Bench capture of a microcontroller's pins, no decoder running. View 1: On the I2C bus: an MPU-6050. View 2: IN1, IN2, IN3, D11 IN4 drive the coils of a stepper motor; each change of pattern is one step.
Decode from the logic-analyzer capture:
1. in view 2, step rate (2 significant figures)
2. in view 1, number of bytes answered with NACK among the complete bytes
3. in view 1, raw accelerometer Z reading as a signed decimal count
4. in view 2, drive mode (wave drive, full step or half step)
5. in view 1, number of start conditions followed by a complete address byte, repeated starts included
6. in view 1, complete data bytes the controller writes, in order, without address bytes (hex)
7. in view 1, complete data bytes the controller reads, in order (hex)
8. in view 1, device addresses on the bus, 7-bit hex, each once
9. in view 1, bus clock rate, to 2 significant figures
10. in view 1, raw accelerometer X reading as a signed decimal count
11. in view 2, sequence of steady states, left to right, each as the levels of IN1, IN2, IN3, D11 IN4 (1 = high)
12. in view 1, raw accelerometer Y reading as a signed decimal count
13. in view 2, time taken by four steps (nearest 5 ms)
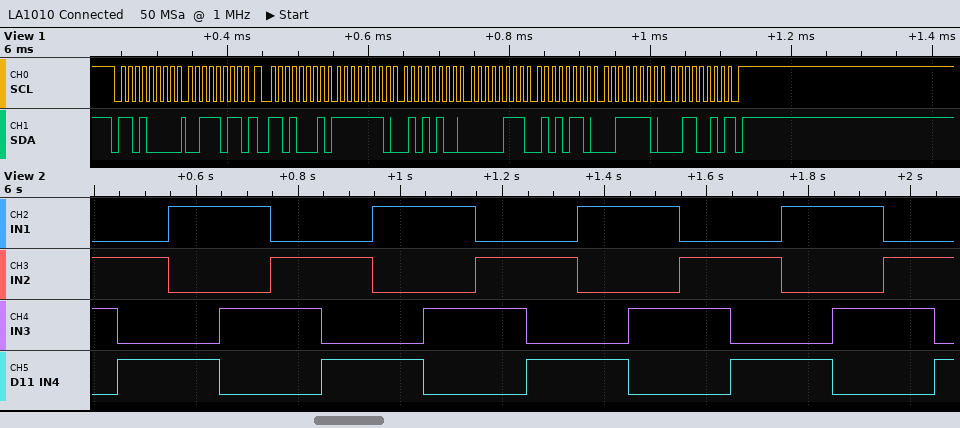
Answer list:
10.0 steps/s
1
15922
full step
2
3B
FE 54 07 56 3E 32
0x68
100 kHz
-428
0110 0101 1001 1010 0110 0101 1001 1010 0110 0101 1001 1010 0110 0101 1001 1010 0110 0101
1878
400 ms
